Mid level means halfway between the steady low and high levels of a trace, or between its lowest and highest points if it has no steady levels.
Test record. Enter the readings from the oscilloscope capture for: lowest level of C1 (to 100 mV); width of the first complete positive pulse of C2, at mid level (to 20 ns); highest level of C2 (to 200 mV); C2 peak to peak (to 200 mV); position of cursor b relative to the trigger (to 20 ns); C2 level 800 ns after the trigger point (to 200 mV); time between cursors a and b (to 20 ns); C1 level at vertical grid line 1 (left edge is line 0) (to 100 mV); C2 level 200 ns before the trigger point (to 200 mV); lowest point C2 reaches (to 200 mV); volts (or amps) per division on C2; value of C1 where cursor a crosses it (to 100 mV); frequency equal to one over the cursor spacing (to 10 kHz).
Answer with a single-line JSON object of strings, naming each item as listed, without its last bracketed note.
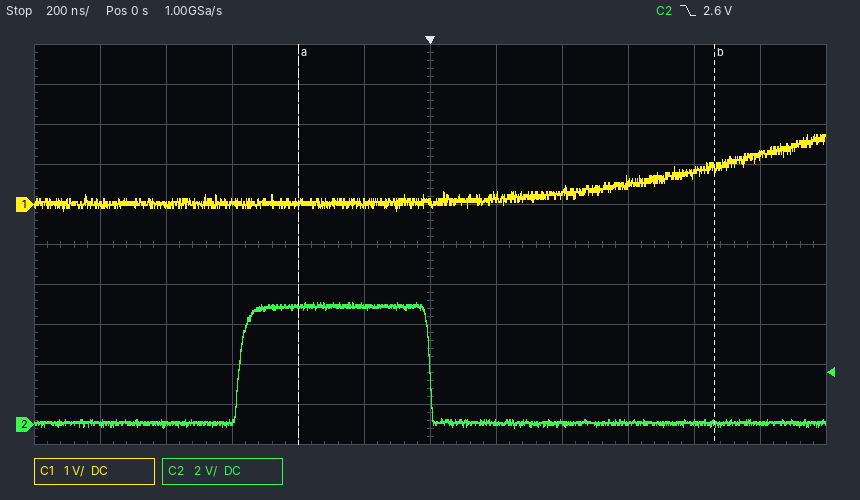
{"lowest level of C1": "-200 mV", "width of the first complete positive pulse of C2, at mid level": "580 ns", "highest level of C2": "6.0 V", "C2 peak to peak": "6.2 V", "position of cursor b relative to the trigger": "+860 ns", "C2 level 800 ns after the trigger point": "200 mV", "time between cursors a and b": "1.26 µs", "C1 level at vertical grid line 1 (left edge is line 0)": "0.0 V", "C2 level 200 ns before the trigger point": "6.0 V", "lowest point C2 reaches": "-200 mV", "volts (or amps) per division on C2": "2 V", "value of C1 where cursor a crosses it": "100 mV", "frequency equal to one over the cursor spacing": "790 kHz"}
